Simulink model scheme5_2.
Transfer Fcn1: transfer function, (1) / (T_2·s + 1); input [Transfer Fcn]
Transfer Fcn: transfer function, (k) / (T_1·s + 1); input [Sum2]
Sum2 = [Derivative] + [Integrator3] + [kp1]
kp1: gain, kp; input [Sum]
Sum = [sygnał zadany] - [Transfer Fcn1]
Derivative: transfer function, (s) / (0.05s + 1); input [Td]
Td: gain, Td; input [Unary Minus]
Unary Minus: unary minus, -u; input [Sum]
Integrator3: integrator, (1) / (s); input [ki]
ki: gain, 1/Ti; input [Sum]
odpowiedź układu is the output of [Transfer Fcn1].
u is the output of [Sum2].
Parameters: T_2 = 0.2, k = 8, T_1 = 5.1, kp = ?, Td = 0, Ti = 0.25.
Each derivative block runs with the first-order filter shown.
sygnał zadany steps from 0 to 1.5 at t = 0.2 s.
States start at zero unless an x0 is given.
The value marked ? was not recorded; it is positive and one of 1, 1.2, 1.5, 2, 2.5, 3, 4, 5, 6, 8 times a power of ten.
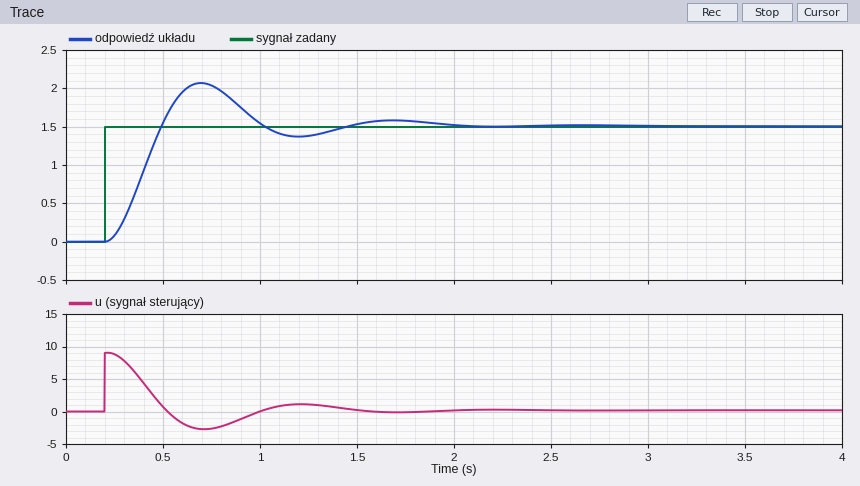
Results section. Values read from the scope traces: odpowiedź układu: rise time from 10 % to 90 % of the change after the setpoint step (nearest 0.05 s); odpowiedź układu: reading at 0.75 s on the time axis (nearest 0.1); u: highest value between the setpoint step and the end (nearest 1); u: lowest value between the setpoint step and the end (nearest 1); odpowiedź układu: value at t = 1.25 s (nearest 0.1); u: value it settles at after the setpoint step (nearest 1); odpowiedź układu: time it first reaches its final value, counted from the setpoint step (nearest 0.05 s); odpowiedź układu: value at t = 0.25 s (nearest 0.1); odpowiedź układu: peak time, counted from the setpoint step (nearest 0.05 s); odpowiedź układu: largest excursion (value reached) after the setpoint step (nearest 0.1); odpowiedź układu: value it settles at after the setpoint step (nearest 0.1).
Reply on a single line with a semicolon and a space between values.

0.20 s; 2.0; 9; -3; 1.4; 0; 0.30 s; 0.1; 0.50 s; 2.1; 1.5
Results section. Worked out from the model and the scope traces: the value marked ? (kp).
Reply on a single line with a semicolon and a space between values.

6
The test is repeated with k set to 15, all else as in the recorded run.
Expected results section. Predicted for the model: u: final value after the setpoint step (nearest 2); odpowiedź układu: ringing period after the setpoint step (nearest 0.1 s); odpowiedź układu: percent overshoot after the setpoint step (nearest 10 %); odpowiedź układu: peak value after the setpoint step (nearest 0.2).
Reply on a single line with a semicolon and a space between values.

0; 0.7 s; 50 %; 2.2
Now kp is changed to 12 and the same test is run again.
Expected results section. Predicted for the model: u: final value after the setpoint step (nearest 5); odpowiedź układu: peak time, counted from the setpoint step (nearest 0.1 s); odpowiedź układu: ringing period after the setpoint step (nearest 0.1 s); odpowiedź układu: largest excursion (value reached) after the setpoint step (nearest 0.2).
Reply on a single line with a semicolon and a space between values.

0; 0.3 s; 0.7 s; 2.2
